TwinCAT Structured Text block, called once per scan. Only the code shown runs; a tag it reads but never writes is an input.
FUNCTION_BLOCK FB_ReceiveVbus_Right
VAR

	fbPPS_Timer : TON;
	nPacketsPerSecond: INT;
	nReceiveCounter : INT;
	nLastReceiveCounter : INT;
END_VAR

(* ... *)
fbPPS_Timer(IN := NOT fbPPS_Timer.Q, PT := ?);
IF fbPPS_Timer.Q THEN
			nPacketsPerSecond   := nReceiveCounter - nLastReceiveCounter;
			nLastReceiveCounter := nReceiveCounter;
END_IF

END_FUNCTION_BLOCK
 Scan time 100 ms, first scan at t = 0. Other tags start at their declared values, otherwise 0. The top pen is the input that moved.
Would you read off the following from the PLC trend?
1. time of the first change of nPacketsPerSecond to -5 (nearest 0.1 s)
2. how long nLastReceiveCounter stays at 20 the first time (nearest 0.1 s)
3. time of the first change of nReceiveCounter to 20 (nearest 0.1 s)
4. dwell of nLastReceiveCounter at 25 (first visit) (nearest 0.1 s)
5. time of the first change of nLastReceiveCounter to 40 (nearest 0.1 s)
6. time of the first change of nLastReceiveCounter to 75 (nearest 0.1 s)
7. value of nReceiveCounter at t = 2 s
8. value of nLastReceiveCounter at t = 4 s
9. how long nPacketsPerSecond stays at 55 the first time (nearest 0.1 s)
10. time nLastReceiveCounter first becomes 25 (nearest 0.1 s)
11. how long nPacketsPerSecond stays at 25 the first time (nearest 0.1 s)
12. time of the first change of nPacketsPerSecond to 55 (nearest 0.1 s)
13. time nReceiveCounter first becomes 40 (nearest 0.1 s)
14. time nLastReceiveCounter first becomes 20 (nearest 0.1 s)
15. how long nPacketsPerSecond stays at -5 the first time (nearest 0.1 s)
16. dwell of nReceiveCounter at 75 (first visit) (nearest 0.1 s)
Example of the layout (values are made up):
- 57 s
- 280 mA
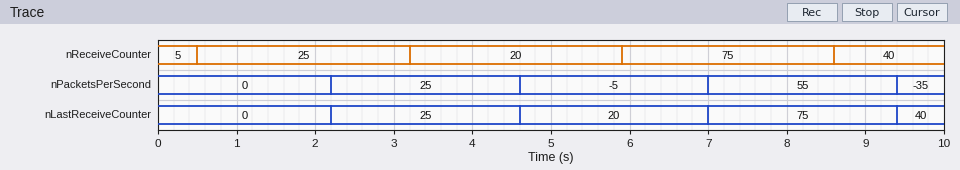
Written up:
- 4.6 s
- 2.4 s
- 3.2 s
- 2.4 s
- 9.4 s
- 7.0 s
- 25
- 25
- 2.4 s
- 2.2 s
- 2.4 s
- 7.0 s
- 8.6 s
- 4.6 s
- 2.4 s
- 2.7 s
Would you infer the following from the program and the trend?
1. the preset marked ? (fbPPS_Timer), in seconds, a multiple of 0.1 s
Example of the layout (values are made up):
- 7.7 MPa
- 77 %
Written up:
- 2.2 s
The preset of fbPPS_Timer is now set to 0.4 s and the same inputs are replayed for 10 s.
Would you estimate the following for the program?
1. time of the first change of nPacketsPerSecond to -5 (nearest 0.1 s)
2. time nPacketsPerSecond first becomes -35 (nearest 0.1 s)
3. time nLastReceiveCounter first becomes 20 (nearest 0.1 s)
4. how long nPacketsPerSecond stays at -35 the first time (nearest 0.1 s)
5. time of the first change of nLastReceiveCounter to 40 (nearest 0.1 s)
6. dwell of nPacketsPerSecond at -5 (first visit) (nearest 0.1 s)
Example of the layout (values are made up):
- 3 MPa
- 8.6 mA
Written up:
- 3.4 s
- 8.8 s
- 3.4 s
- 0.6 s
- 8.8 s
- 0.6 s
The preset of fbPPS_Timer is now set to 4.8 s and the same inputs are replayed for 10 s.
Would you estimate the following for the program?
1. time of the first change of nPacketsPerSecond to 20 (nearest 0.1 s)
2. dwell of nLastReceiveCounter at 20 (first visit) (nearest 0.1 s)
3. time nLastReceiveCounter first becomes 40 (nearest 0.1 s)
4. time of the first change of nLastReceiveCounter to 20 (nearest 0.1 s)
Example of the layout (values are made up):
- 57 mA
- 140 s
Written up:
- 4.8 s
- 5.0 s
- 9.8 s
- 4.8 s
